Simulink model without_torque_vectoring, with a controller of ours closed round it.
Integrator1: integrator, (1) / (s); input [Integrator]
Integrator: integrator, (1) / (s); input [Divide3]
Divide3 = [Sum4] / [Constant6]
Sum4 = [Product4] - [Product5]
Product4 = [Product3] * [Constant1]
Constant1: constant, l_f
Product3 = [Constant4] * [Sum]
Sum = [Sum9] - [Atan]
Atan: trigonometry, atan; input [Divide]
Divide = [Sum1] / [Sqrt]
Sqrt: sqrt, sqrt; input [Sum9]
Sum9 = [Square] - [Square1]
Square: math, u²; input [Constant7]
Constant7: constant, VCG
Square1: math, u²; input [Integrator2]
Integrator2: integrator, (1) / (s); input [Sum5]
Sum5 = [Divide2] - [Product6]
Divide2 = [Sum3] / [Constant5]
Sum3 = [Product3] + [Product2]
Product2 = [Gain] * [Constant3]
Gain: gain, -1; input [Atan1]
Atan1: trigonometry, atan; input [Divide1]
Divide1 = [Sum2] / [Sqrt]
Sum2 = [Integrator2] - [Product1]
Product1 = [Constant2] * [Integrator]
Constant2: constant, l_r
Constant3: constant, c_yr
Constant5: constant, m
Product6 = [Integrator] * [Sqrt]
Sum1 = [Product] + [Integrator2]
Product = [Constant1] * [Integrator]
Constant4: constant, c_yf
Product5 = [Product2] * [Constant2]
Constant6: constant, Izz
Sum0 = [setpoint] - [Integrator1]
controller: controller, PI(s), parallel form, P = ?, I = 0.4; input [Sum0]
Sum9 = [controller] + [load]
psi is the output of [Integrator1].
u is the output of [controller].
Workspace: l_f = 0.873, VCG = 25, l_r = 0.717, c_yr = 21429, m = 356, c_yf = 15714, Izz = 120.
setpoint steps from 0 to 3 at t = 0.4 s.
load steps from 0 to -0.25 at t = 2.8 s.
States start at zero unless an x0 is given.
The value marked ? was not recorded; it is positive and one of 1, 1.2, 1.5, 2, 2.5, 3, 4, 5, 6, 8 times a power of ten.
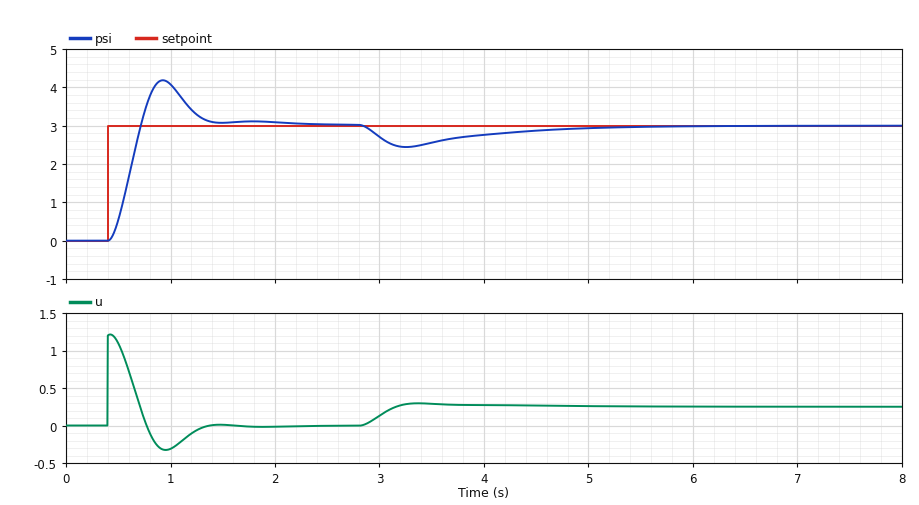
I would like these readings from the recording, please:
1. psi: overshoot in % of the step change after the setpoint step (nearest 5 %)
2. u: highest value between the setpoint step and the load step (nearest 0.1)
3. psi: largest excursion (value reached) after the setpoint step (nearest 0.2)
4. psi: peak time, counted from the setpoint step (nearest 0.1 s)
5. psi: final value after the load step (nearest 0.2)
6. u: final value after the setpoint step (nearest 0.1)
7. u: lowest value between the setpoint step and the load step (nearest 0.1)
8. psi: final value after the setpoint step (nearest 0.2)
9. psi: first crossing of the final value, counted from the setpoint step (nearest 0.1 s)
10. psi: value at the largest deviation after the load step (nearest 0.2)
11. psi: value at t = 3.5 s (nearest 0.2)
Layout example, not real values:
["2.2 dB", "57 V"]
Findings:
["40 %", "1.2", "4.2", "0.5 s", "3.0", "0.0", "-0.3", "3.0", "0.3 s", "2.4", "2.6"]
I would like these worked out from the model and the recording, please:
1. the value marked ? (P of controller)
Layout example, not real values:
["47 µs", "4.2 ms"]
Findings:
["0.4"]
